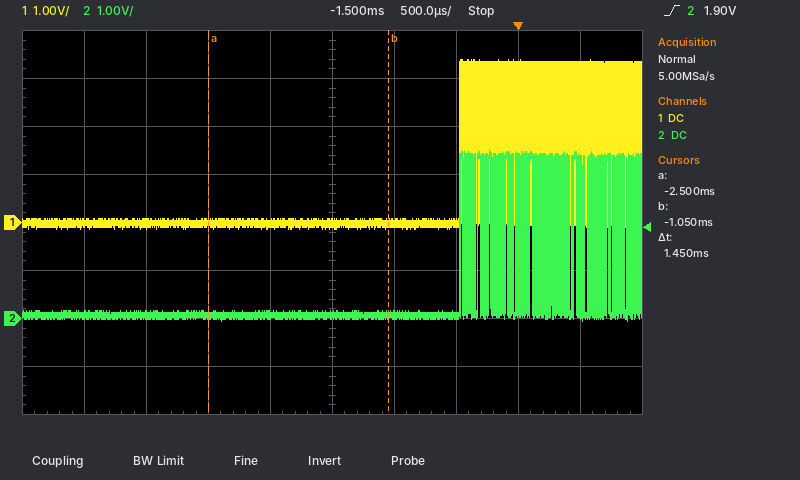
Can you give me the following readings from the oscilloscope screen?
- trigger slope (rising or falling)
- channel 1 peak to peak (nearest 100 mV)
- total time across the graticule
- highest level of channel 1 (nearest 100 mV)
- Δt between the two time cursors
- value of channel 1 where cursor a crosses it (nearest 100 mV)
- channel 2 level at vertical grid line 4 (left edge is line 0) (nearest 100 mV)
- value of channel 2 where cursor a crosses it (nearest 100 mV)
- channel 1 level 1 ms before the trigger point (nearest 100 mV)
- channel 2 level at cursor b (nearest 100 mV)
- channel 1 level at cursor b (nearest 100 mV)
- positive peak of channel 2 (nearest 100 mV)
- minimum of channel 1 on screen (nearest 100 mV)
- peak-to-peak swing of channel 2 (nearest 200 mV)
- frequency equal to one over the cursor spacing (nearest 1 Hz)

rising
3.5 V
5 ms
3.4 V
1.45 ms
0.0 V
100 mV
100 mV
0.0 V
100 mV
0.0 V
3.5 V
-100 mV
3.6 V
690 Hz
